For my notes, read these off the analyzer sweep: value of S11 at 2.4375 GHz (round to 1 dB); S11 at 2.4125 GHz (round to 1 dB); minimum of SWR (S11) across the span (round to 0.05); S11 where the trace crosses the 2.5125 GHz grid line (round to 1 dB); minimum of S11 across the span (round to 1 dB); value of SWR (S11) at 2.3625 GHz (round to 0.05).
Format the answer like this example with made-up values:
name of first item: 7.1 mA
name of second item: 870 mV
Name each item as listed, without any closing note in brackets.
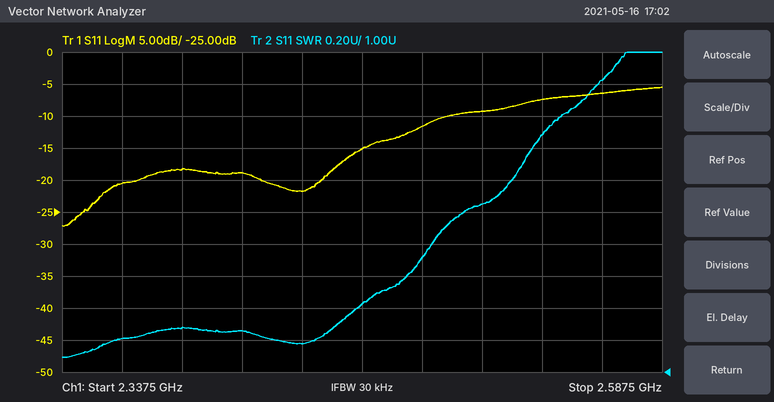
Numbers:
value of S11 at 2.4375 GHz: -22 dB
S11 at 2.4125 GHz: -19 dB
minimum of SWR (S11) across the span: 1.10
S11 where the trace crosses the 2.5125 GHz grid line: -9 dB
minimum of S11 across the span: -27 dB
value of SWR (S11) at 2.3625 GHz: 1.20
